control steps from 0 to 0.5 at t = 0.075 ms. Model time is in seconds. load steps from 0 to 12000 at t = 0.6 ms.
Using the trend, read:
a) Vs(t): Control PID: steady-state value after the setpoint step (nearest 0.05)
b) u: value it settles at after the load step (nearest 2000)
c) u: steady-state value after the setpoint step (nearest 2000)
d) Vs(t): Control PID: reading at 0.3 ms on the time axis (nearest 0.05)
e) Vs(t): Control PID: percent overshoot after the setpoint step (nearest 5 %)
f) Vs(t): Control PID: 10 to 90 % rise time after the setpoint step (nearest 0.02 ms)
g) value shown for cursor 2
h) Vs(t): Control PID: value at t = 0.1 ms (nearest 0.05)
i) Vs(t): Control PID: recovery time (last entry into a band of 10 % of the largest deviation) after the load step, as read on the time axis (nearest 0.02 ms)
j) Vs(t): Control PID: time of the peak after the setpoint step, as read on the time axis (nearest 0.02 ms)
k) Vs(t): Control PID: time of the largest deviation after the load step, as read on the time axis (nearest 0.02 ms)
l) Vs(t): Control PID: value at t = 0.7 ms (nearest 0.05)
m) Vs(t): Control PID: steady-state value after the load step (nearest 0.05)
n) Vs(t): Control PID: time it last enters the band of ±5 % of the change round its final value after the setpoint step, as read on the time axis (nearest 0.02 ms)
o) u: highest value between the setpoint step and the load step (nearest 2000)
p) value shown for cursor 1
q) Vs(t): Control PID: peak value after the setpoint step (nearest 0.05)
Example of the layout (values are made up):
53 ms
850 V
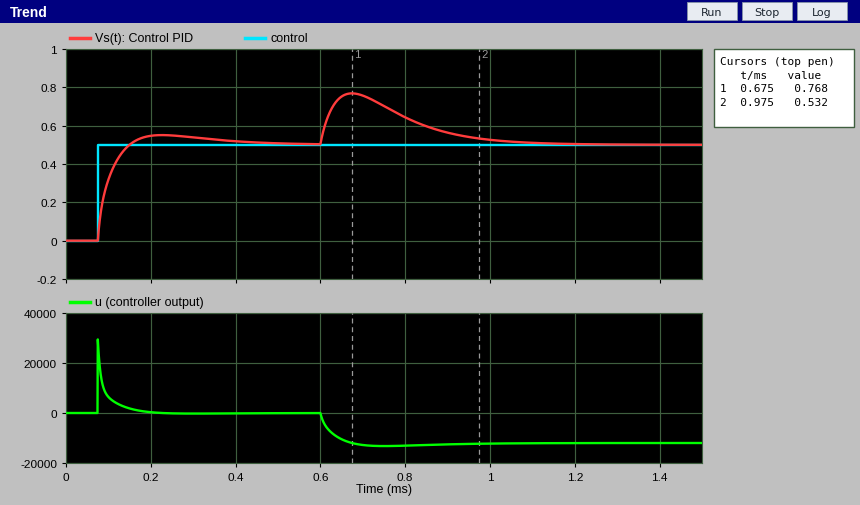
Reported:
0.50
-12000
0
0.55
10 %
0.06 ms
0.532
0.30
1.00 ms
0.22 ms
0.68 ms
0.75
0.50
0.36 ms
30000
0.768
0.55
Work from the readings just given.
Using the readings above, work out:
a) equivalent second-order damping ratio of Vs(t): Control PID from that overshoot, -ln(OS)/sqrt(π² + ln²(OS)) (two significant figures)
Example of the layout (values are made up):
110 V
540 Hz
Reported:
0.59
